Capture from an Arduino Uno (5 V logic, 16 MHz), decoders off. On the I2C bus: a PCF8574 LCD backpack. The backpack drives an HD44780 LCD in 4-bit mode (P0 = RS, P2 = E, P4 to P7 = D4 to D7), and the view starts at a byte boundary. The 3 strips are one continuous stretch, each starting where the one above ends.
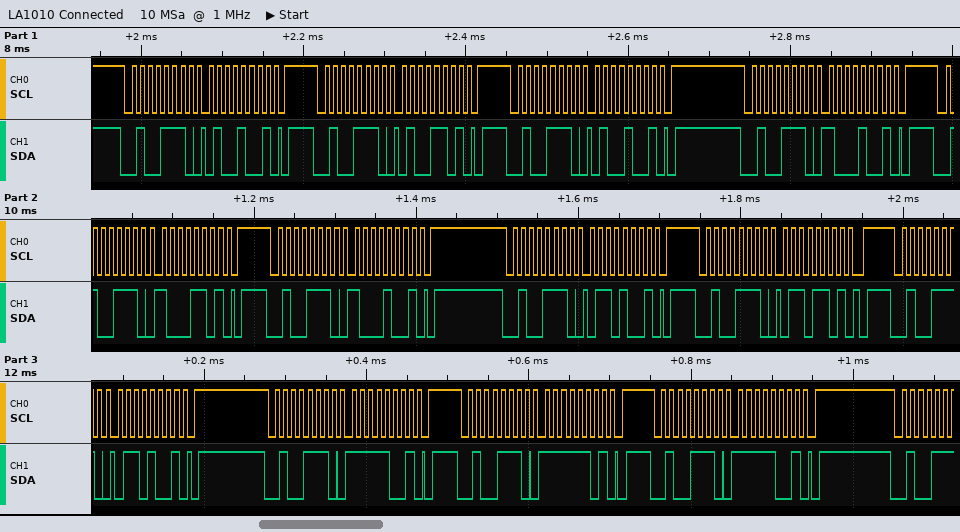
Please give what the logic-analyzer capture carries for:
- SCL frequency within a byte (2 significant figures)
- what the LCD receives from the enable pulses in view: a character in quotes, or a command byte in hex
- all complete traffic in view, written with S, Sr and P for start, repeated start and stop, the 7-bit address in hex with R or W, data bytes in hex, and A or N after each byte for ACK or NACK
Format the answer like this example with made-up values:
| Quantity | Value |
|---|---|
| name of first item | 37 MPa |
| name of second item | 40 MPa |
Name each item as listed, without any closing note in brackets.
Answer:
| Quantity | Value |
|---|---|
| SCL frequency within a byte | 100 kHz |
| what the LCD receives from the enable pulses in view: a character in quotes, or a command byte in hex | 'H' 'o' |
| all complete traffic in view, written with S, Sr and P for start, repeated start and stop, the 7-bit address in hex with R or W, data bytes in hex, and A or N after each byte for ACK or NACK | S 27W A 49 A P S 27W A 4D A P S 27W A 49 A P S 27W A 89 A P S 27W A 8D A P S 27W A 89 A P S 27W A 69 A P S 27W A 6D A P S 27W A 69 A P S 27W A F9 A P S 27W A FD A P S 27W A F9 A P |
